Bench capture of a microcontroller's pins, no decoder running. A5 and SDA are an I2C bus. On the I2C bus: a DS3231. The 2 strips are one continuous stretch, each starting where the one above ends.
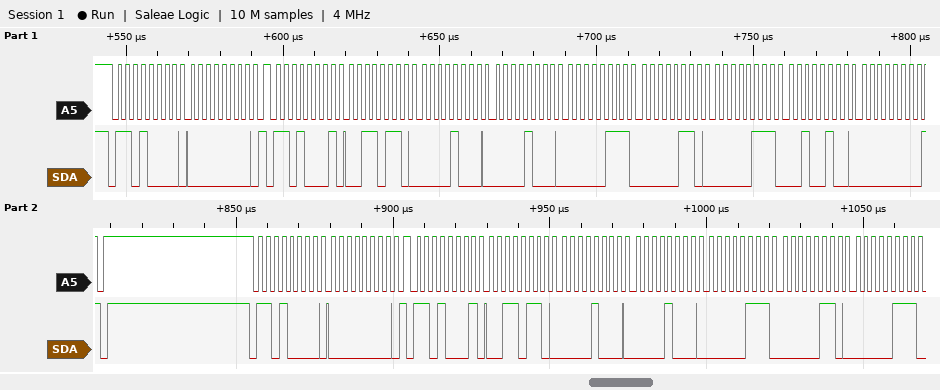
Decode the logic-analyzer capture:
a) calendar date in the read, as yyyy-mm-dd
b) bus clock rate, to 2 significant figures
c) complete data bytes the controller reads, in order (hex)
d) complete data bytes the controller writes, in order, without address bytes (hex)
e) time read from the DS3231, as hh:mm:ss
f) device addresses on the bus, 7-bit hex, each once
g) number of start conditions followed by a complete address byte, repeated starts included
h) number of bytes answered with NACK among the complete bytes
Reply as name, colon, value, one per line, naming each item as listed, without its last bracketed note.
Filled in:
calendar date in the read, as yyyy-mm-dd: 2024-07-06
bus clock rate, to 2 significant figures: 400 kHz
complete data bytes the controller reads, in order: 36 08 08 07 06 07 24 00 36 08 08 07 06 07
complete data bytes the controller writes, in order, without address bytes: 00 00
time read from the DS3231, as hh:mm:ss: 08:08:36
device addresses on the bus, 7-bit hex, each once: 0x68
number of start conditions followed by a complete address byte, repeated starts included: 4
number of bytes answered with NACK among the complete bytes: 1
